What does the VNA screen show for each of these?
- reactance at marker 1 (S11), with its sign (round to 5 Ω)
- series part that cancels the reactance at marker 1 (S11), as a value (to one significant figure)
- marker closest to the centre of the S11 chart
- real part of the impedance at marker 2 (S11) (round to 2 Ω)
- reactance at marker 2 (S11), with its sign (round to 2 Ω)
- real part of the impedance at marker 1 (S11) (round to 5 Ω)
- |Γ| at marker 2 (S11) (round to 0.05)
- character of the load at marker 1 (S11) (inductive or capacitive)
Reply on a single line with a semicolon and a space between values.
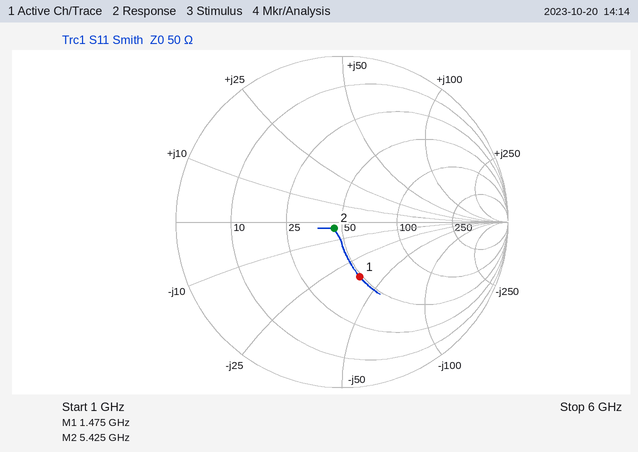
-35 Ω; 4 nH; marker 2; 46 Ω; -4 Ω; 50 Ω; 0.05; capacitive
